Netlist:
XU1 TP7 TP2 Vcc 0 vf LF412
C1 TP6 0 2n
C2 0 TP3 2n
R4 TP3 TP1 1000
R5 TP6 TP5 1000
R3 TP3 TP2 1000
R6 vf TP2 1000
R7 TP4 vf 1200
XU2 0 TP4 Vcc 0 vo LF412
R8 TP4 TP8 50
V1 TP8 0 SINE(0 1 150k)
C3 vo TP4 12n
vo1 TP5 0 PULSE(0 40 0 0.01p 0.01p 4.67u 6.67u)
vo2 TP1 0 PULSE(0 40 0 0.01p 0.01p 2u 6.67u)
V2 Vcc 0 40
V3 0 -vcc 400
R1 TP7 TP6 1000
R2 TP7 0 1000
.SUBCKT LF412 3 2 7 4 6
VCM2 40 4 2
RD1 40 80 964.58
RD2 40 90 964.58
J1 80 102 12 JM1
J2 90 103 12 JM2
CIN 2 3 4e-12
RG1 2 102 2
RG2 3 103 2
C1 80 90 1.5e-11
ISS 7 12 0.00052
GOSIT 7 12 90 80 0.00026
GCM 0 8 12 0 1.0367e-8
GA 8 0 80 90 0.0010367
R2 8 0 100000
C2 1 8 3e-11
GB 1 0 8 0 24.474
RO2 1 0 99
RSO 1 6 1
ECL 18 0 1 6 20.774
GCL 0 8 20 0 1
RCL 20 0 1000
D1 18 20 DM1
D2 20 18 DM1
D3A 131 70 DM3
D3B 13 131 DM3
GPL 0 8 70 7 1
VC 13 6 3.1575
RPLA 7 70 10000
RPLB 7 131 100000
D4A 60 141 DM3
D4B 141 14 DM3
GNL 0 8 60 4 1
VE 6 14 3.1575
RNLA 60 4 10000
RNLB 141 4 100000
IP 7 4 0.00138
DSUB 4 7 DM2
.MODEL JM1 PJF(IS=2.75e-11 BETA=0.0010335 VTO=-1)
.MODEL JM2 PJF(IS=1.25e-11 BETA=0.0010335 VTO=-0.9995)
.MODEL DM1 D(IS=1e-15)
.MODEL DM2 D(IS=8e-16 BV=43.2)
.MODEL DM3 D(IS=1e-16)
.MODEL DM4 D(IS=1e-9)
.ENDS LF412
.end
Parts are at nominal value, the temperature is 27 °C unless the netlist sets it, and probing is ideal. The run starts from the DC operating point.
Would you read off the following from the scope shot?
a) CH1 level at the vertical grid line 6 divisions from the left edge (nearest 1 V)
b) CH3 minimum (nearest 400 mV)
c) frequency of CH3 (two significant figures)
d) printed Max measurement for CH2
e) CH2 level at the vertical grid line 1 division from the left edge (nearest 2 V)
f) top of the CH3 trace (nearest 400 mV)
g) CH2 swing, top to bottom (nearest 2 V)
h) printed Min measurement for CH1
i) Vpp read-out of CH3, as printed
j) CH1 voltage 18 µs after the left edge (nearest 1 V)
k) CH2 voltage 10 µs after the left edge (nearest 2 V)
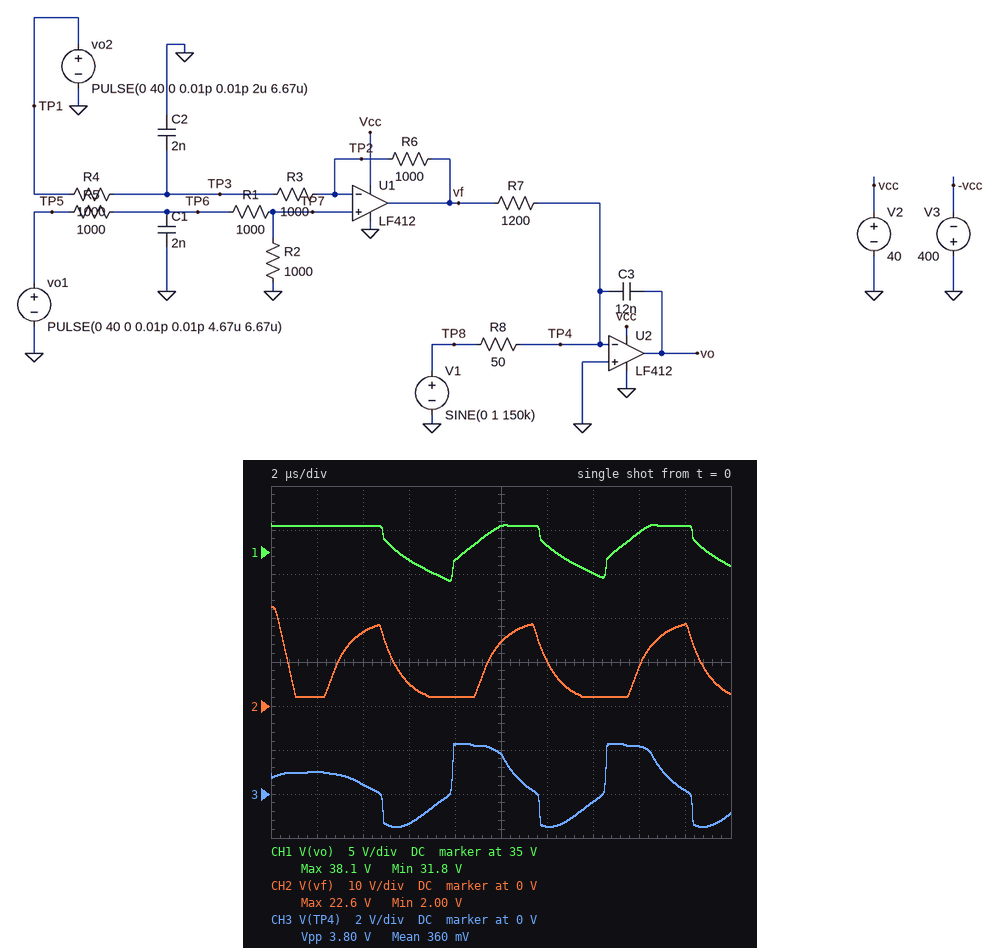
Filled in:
36 V
-1.6 V
150 kHz
22.6 V
2 V
2.4 V
20 V
31.8 V
3.80 V
38 V
14 V
